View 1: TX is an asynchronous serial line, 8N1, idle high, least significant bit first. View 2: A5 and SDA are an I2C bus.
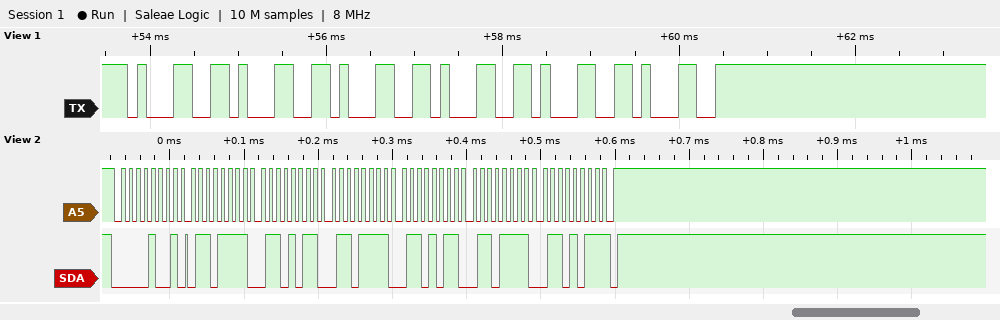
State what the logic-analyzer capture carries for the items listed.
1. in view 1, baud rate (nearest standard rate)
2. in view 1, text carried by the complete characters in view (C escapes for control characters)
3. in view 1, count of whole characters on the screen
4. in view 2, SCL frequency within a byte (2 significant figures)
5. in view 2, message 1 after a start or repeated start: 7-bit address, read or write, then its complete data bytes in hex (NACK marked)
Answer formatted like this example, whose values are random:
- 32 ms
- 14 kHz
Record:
- 9600 baud
- "111111"
- 6
- 100 kHz
- 0x04 read: 6F 6B 6F 6B 6F 6B NACK
